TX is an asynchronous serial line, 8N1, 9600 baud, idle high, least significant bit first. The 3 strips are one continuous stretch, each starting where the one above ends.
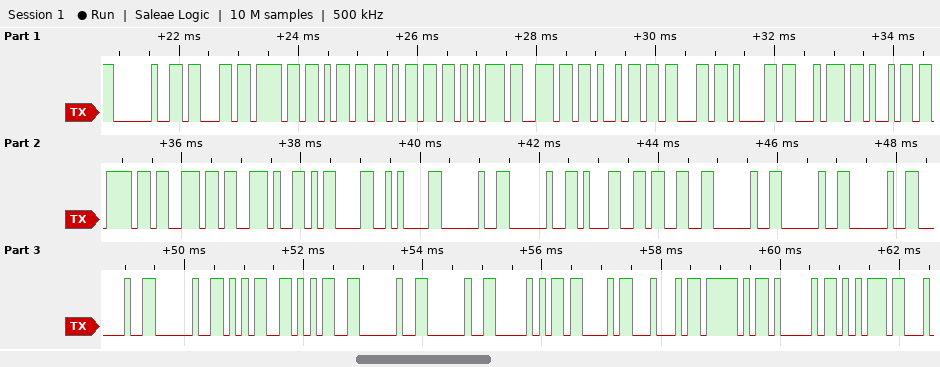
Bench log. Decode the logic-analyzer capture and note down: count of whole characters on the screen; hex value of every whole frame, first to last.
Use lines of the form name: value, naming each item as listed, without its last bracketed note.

count of whole characters on the screen: 36
hex value of every whole frame, first to last: 0x20 0x63 0x6F 0x6D 0x6D 0x75 0x6E 0x69 0x63 0x61 0x74 0x69 0x6F 0x6E 0x2E 0x0D 0x0A 0x20 0x20 0x31 0x33 0x20 0x20 0x20 0x20 0x20 0x35 0x35 0x20 0x20 0x50 0x43 0x44 0x5F 0x41 0x75
